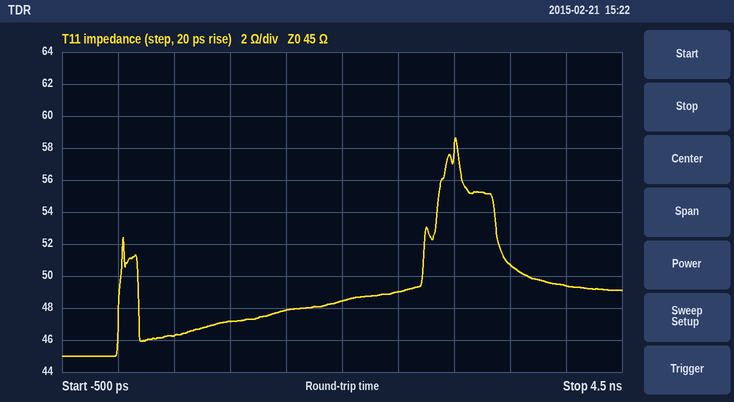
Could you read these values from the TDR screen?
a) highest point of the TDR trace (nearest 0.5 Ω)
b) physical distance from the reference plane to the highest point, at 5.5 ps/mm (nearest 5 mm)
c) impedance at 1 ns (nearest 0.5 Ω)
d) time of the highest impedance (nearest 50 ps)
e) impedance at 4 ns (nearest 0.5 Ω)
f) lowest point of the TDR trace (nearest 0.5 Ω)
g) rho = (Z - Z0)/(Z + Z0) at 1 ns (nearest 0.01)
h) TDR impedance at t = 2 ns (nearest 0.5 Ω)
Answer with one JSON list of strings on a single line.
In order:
["58.5 Ω", "275 mm", "47.0 Ω", "3.00 ns", "49.5 Ω", "45.0 Ω", "+0.02", "48.5 Ω"]
